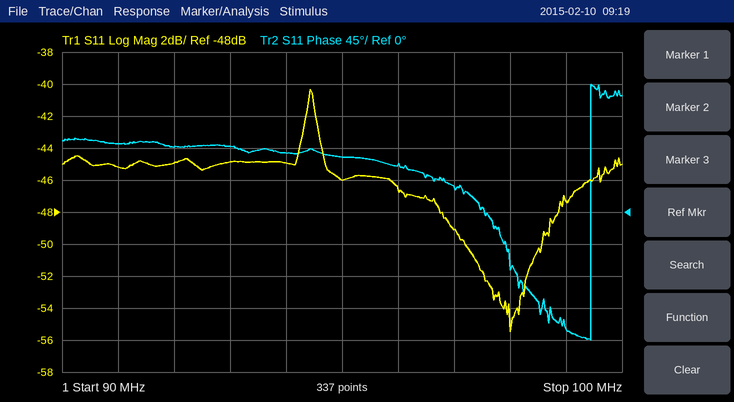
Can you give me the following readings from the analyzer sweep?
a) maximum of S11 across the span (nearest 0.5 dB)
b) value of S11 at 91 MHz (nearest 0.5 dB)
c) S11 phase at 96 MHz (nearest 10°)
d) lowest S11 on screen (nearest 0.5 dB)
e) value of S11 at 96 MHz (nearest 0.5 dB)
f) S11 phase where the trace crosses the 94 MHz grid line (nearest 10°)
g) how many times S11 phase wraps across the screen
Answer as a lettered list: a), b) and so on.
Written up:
a) -40.5 dB
b) -45.0 dB
c) 70°
d) -55.5 dB
e) -46.5 dB
f) 80°
g) 1
